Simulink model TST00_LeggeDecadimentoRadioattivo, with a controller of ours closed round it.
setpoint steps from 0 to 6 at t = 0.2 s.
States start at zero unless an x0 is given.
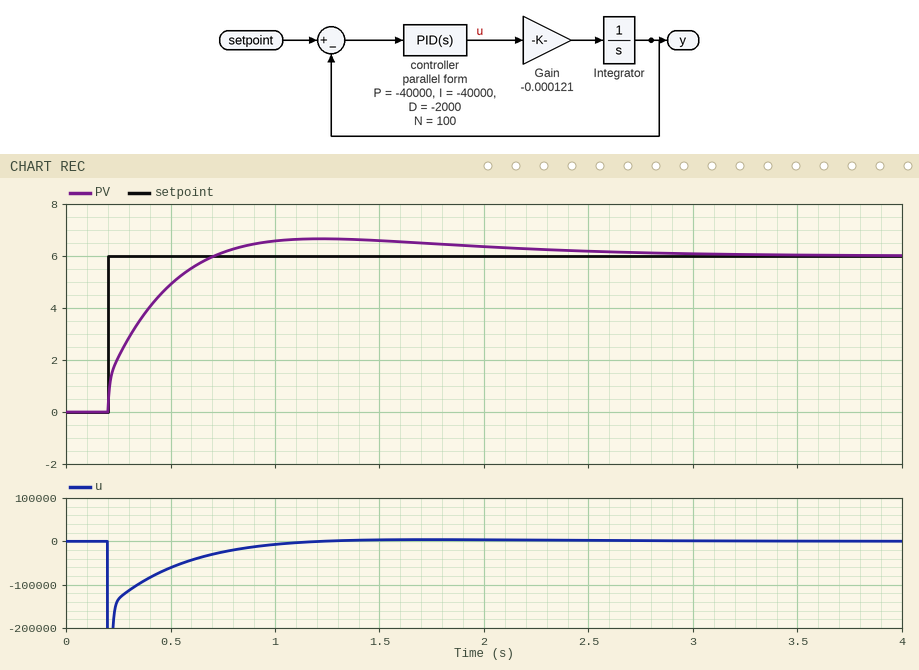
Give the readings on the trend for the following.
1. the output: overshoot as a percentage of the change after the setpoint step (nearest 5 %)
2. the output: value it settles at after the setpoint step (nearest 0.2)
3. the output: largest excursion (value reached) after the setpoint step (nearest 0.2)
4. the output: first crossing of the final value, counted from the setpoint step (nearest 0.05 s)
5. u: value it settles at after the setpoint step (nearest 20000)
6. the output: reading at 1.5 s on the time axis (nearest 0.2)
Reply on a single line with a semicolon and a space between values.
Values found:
10 %; 6.0; 6.6; 0.50 s; 0; 6.6
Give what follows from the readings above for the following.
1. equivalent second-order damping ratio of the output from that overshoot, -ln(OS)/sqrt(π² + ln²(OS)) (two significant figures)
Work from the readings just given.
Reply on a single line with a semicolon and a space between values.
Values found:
0.59
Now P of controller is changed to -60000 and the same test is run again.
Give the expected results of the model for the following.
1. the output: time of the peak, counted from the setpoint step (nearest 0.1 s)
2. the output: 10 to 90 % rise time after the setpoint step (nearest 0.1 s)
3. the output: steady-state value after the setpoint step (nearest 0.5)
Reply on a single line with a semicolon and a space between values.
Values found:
0.9 s; 0.3 s; 6.0
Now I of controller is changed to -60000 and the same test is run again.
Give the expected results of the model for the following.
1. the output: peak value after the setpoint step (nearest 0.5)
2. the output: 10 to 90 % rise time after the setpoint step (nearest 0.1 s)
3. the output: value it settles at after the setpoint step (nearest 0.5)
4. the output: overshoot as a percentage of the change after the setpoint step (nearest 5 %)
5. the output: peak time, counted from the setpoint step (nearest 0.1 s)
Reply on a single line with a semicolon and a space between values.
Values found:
7.0; 0.3 s; 6.0; 15 %; 0.9 s
